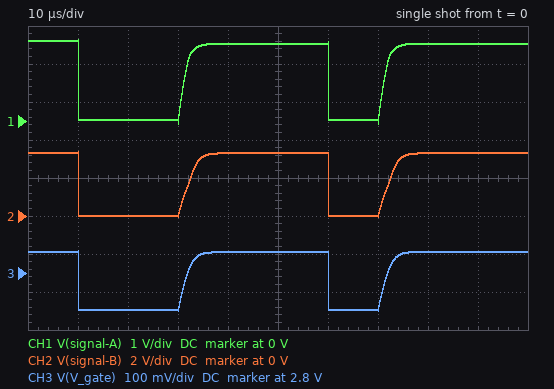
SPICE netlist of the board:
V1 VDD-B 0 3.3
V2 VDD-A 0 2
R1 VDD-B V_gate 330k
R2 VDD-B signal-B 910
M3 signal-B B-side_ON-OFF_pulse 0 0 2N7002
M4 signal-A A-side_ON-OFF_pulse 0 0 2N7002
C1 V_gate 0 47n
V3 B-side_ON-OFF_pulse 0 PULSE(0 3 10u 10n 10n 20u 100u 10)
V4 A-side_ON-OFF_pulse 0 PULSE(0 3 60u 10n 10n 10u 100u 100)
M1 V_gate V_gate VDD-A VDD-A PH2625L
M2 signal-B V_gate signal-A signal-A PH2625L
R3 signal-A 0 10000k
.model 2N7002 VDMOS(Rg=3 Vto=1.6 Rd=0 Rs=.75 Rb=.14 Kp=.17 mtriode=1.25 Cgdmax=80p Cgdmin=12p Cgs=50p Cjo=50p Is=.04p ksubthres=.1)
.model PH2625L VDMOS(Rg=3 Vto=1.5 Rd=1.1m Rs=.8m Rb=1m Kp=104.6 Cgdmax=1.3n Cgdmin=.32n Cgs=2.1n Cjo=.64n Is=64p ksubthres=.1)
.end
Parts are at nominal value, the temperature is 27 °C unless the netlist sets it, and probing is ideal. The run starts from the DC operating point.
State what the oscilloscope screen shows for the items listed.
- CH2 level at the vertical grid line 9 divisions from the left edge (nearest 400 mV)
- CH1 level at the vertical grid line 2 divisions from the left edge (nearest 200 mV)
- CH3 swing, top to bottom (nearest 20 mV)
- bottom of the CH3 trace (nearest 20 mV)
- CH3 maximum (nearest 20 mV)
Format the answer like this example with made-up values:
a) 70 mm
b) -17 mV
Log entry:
a) 3.2 V
b) 0 V
c) 160 mV
d) 2.70 V
e) 2.86 V
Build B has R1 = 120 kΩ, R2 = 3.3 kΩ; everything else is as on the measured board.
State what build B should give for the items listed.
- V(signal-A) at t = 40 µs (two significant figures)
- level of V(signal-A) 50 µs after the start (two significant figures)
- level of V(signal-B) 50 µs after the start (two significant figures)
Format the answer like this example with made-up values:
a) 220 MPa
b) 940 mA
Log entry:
a) 1.9 V
b) 2.1 V
c) 3.2 V
